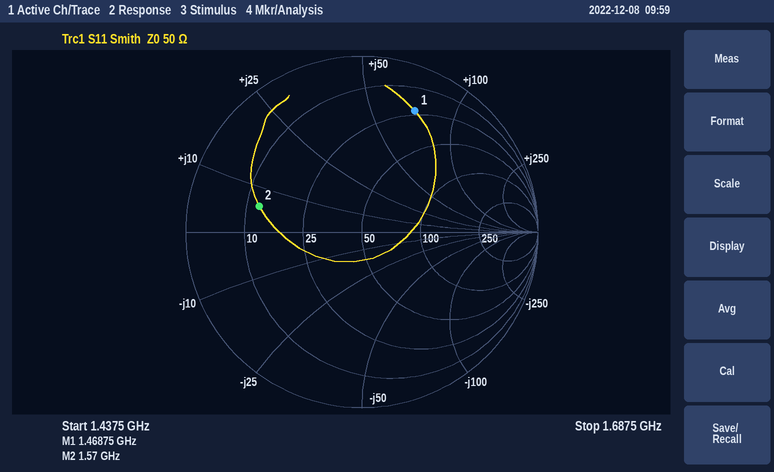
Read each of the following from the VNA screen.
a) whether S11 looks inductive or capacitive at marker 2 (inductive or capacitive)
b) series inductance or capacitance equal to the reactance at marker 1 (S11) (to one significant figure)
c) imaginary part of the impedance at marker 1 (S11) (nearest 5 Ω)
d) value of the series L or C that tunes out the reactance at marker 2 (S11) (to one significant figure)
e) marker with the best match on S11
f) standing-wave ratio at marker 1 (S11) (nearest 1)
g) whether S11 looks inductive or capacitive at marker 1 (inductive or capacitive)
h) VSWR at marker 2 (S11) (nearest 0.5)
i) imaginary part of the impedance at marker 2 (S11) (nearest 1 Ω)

inductive
8 nH
+70 Ω
20 pF
marker 2
7
inductive
4.0
+6 Ω
